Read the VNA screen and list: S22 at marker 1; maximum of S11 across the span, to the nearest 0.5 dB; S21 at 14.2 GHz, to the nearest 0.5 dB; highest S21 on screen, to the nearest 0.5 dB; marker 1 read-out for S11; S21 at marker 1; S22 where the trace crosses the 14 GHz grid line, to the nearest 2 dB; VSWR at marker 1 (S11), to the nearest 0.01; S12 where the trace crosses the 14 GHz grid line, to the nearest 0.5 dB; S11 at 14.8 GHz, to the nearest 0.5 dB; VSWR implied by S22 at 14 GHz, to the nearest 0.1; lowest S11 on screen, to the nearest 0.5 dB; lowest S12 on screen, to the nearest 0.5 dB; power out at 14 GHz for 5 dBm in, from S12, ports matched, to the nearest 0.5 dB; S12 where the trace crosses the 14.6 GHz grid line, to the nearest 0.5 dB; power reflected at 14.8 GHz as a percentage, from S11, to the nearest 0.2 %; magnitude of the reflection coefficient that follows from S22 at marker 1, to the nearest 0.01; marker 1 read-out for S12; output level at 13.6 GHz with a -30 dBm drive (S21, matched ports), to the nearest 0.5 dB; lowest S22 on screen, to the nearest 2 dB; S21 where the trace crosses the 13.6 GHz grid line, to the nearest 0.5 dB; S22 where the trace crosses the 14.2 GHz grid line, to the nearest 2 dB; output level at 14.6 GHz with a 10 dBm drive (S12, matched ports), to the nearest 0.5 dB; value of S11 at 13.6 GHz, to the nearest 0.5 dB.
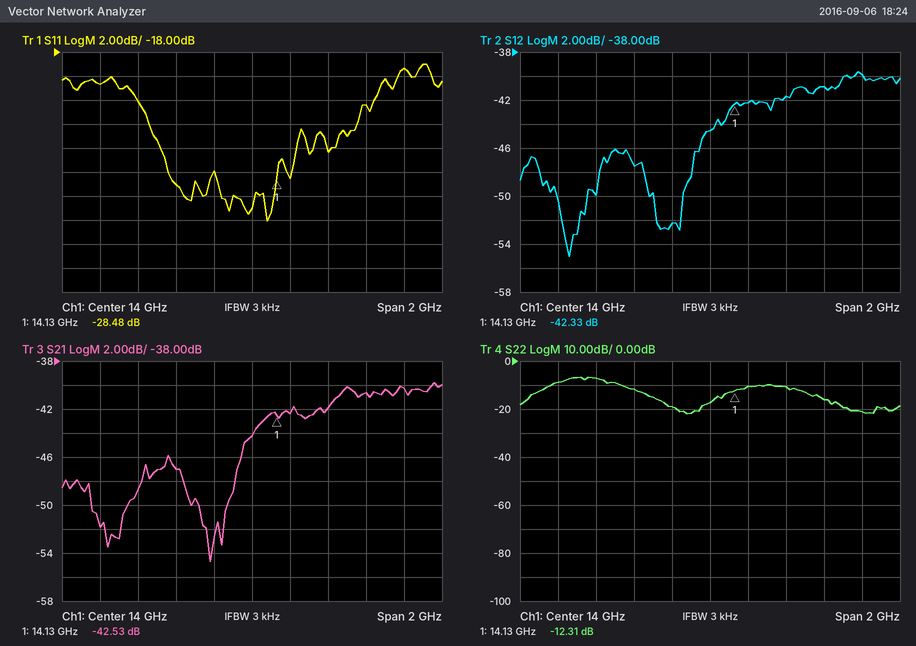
-12.31 dB
-19.0 dB
-42.5 dB
-40.0 dB
-28.48 dB
-42.53 dB
-18 dB
1.08
-44.5 dB
-19.5 dB
1.3
-32.0 dB
-55.0 dB
-39.5 dBm
-41.0 dB
1.2 %
0.24
-42.33 dB
-77.0 dBm
-22 dB
-47.0 dB
-10 dB
-31.0 dBm
-29.0 dB
